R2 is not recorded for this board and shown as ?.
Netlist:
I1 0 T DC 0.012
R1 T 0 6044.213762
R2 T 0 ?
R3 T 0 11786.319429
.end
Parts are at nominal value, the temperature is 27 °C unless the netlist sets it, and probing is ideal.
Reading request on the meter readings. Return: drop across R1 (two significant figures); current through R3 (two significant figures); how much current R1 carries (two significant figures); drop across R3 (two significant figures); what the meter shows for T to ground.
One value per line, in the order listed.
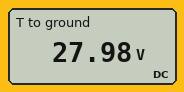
28 V
2.4 mA
4.6 mA
28 V
27.98 V
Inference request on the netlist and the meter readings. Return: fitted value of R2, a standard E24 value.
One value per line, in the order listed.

5.6 kΩ
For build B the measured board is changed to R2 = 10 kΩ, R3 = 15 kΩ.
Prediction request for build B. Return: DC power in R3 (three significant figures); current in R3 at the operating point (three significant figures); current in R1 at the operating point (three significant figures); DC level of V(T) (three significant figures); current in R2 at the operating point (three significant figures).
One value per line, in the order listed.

87.0 mW
2.41 mA
5.98 mA
36.1 V
3.61 mA
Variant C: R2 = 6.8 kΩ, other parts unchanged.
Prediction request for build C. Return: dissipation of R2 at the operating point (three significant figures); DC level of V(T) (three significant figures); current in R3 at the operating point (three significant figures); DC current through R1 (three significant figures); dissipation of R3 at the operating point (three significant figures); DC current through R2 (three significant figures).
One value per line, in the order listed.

134 mW
30.2 V
2.56 mA
5.00 mA
77.4 mW
4.44 mA
